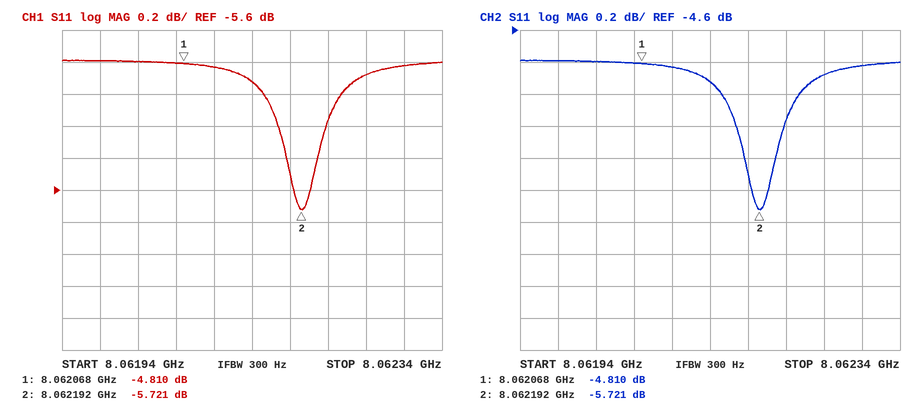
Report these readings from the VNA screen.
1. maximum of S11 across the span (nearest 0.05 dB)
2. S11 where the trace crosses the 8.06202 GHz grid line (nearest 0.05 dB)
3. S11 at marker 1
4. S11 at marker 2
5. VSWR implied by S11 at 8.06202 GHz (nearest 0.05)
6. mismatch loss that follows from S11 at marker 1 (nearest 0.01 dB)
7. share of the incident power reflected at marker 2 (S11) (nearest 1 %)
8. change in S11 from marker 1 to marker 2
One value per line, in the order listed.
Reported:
-4.80 dB
-4.80 dB
-4.810 dB
-5.721 dB
3.70
1.74 dB
27 %
-0.911 dB
